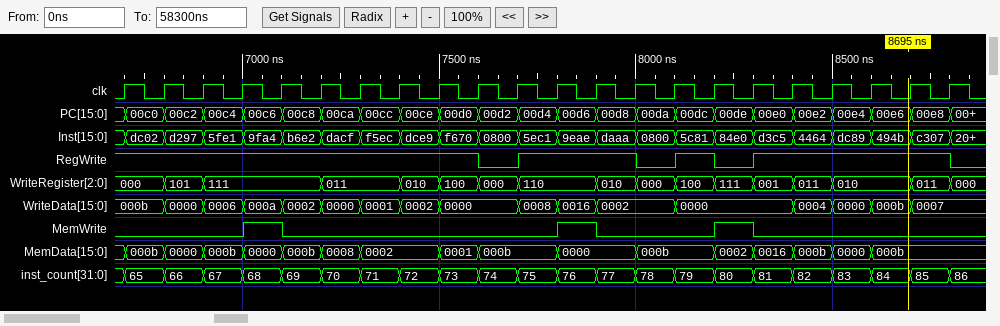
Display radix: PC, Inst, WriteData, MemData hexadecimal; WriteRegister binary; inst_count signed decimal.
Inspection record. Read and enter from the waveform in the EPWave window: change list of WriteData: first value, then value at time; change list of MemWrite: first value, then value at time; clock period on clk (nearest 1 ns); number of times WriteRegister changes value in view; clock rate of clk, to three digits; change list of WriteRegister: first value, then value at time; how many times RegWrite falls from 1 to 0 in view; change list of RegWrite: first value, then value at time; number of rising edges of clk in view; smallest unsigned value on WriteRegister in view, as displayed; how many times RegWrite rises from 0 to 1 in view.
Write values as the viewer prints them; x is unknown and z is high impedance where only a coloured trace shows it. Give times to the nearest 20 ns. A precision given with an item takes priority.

000b, 0000 at 6800 ns, 0006 at 6900 ns, 000a at 7000 ns, 0002 at 7100 ns, 0000 at 7200 ns, 0001 at 7300 ns, 0002 at 7400 ns, 0000 at 7500 ns, 0008 at 7700 ns, 0016 at 7800 ns, 0002 at 7900 ns, 0000 at 8100 ns, 0004 at 8400 ns, 0000 at 8500 ns, 000b at 8600 ns, 0007 at 8700 ns
0, 1 at 7000 ns, 0 at 7100 ns, 1 at 7800 ns, 0 at 7900 ns, 1 at 8200 ns, 0 at 8300 ns
100 ns
16
10.0 MHz
000, 101 at 6800 ns, 111 at 6900 ns, 011 at 7200 ns, 010 at 7400 ns, 100 at 7500 ns, 000 at 7600 ns, 110 at 7700 ns, 010 at 7900 ns, 000 at 8000 ns, 100 at 8100 ns, 111 at 8200 ns, 001 at 8300 ns, 011 at 8400 ns, 010 at 8500 ns, 011 at 8700 ns, 000 at 8800 ns
4
1, 0 at 7600 ns, 1 at 7700 ns, 0 at 8000 ns, 1 at 8100 ns, 0 at 8200 ns, 1 at 8300 ns, 0 at 8800 ns
22
000
3
